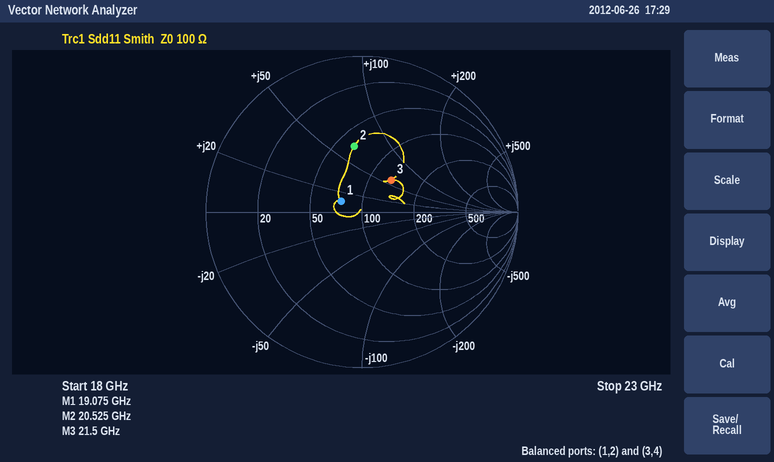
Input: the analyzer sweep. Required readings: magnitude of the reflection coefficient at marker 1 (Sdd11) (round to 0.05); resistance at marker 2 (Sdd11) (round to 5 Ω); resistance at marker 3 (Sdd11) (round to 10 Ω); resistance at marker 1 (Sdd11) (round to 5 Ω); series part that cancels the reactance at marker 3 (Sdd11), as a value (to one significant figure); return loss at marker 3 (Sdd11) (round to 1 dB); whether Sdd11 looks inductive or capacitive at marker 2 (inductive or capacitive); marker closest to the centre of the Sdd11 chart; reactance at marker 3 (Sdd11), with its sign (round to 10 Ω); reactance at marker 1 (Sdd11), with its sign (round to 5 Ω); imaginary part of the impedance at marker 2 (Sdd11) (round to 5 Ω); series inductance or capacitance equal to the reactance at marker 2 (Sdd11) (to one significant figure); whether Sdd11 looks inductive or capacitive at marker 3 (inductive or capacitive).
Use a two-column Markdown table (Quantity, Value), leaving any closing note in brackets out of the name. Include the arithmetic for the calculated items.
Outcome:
| Quantity | Value |
|---|---|
| magnitude of the reflection coefficient at marker 1 (Sdd11) | 0.15 |
| resistance at marker 2 (Sdd11) | 65 Ω |
| resistance at marker 3 (Sdd11) | 130 Ω |
| resistance at marker 1 (Sdd11) | 75 Ω |
| series part that cancels the reactance at marker 3 (Sdd11), as a value | C = 1/(2π × 21.5 GHz × 60 Ω) ≈ 123 fF, so 100 fF to one significant figure |
| return loss at marker 3 (Sdd11) | 11 dB |
| whether Sdd11 looks inductive or capacitive at marker 2 | inductive |
| marker closest to the centre of the Sdd11 chart | marker 1 |
| reactance at marker 3 (Sdd11), with its sign | +60 Ω |
| reactance at marker 1 (Sdd11), with its sign | +10 Ω |
| imaginary part of the impedance at marker 2 (Sdd11) | +65 Ω |
| series inductance or capacitance equal to the reactance at marker 2 (Sdd11) | L = 65 Ω/(2π × 20.525 GHz) ≈ 504 pH, so 500 pH to one significant figure |
| whether Sdd11 looks inductive or capacitive at marker 3 | inductive |
